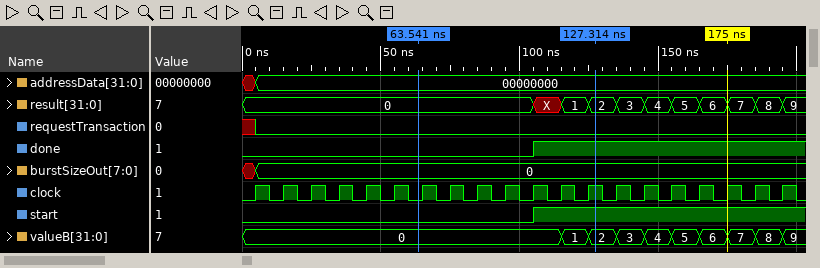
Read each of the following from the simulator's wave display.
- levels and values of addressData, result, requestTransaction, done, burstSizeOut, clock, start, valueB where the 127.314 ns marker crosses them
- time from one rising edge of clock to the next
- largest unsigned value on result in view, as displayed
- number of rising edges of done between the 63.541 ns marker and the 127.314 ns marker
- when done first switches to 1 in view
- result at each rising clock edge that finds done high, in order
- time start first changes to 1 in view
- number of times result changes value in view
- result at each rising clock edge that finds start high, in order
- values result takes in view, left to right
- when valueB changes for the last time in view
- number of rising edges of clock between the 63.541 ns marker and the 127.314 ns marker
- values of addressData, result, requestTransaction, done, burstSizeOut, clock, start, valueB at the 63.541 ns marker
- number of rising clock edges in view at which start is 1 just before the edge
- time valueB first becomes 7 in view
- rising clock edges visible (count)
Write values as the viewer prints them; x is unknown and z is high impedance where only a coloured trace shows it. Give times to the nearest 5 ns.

addressData=00000000, result=2, requestTransaction=0, done=1, burstSizeOut=0, clock=1, start=1, valueB=2
10 ns
9
1
105 ns
X, 1, 2, 3, 4, 5, 6, 7, 8
105 ns
10
X, 1, 2, 3, 4, 5, 6, 7, 8
0, X, 1, 2, 3, 4, 5, 6, 7, 8, 9
195 ns
7
addressData=00000000, result=0, requestTransaction=0, done=0, burstSizeOut=0, clock=0, start=0, valueB=0
9
175 ns
20
